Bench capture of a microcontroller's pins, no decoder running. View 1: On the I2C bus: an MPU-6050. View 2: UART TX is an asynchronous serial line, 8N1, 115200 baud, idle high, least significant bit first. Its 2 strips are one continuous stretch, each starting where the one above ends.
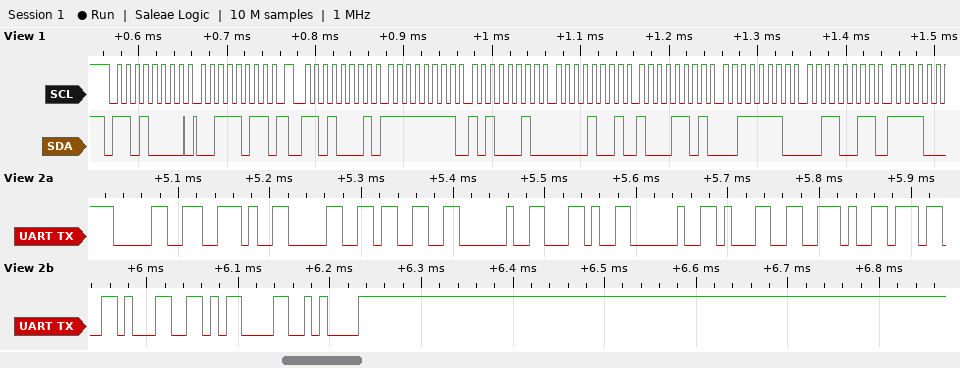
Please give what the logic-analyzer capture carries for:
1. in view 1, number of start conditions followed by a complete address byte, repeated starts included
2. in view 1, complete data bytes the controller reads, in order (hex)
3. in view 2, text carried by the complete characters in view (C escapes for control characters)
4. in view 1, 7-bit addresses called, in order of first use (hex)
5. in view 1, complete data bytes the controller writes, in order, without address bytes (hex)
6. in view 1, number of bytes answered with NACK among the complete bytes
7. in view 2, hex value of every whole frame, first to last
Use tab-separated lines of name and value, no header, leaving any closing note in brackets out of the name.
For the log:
in view 1, number of start conditions followed by a complete address byte, repeated starts included	2
in view 1, complete data bytes the controller reads, in order	FF A2 09 8D 3E 33
in view 2, text carried by the complete characters in view	"0.03 , 1.71\r\n"
in view 1, 7-bit addresses called, in order of first use	0x68
in view 1, complete data bytes the controller writes, in order, without address bytes	3B
in view 1, number of bytes answered with NACK among the complete bytes	0
in view 2, hex value of every whole frame, first to last	0x30 0x2E 0x30 0x33 0x20 0x2C 0x20 0x31 0x2E 0x37 0x31 0x0D 0x0A
